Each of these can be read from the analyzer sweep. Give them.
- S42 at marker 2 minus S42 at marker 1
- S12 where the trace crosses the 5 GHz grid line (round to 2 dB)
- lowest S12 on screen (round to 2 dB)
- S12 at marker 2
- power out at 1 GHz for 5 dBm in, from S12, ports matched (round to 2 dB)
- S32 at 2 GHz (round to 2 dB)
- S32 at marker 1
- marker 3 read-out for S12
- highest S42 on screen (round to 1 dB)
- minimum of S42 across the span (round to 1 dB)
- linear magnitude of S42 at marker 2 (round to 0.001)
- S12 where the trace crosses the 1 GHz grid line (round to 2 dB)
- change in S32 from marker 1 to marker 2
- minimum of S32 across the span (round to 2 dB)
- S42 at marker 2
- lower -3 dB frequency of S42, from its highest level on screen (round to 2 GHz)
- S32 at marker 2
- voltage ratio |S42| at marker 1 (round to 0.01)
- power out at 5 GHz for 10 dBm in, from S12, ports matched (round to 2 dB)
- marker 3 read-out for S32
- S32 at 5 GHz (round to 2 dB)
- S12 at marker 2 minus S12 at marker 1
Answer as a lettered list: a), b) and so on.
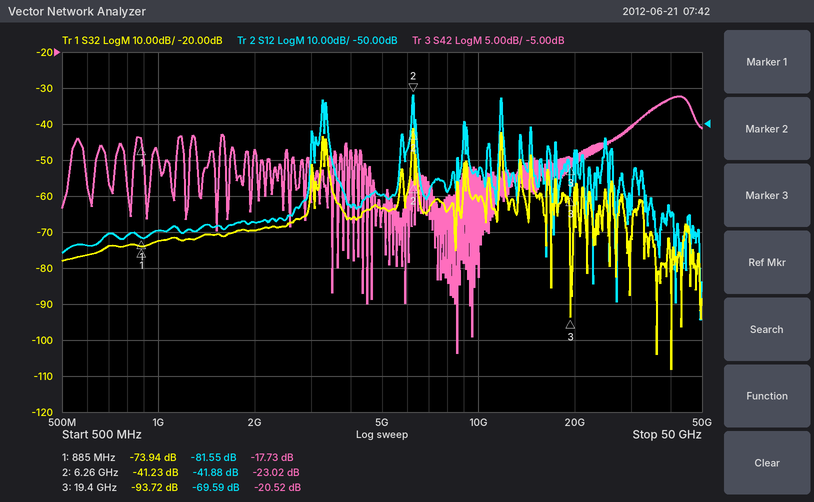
a) -5.29 dB
b) -70 dB
c) -104 dB
d) -41.88 dB
e) -74 dBm
f) -70 dB
g) -73.94 dB
h) -69.59 dB
i) -11 dB
j) -47 dB
k) 0.071
l) -80 dB
m) 32.71 dB
n) -108 dB
o) -23.02 dB
p) 32 GHz
q) -41.23 dB
r) 0.13
s) -60 dBm
t) -93.72 dB
u) -64 dB
v) 39.67 dB
